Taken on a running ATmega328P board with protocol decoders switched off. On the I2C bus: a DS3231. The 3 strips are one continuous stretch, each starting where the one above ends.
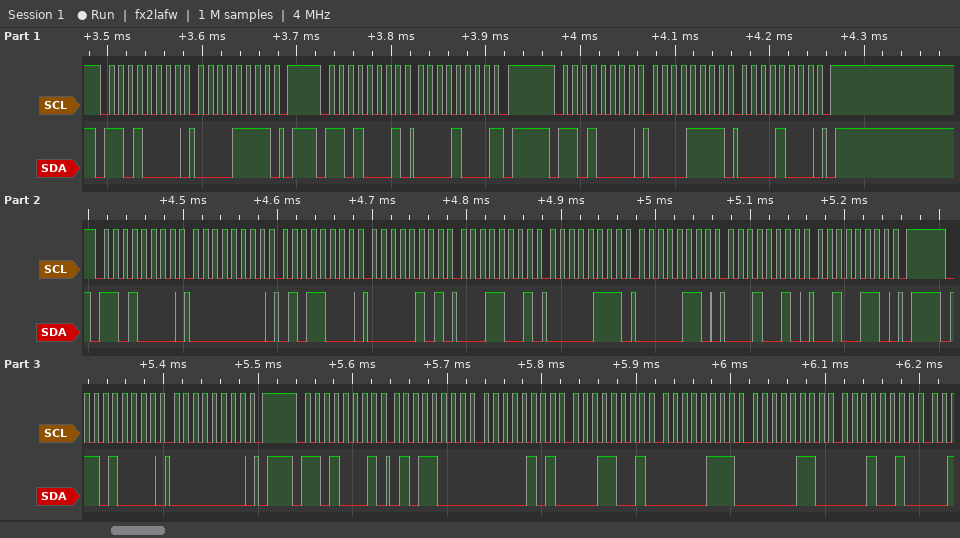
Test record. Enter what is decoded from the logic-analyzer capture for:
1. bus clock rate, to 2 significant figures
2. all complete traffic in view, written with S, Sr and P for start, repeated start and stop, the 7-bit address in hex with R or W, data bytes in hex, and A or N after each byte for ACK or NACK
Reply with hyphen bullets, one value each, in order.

- 100 kHz
- S 68W A 0F A P S 68R A 08 N P S 68W A 0F A 08 A P S 68W A 00 A 58 A 05 A 19 A 07 A 06 A 12 A 26 A P S 68W A 00 A P S 68R A 58 A 05 A 19 A 07 A 06 A 12 A
